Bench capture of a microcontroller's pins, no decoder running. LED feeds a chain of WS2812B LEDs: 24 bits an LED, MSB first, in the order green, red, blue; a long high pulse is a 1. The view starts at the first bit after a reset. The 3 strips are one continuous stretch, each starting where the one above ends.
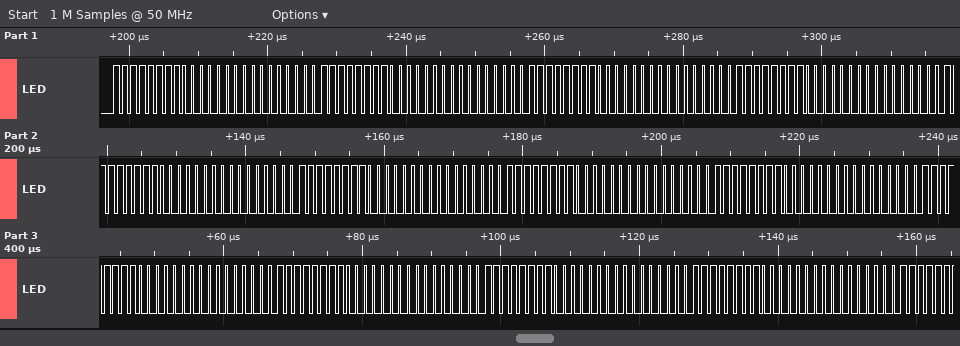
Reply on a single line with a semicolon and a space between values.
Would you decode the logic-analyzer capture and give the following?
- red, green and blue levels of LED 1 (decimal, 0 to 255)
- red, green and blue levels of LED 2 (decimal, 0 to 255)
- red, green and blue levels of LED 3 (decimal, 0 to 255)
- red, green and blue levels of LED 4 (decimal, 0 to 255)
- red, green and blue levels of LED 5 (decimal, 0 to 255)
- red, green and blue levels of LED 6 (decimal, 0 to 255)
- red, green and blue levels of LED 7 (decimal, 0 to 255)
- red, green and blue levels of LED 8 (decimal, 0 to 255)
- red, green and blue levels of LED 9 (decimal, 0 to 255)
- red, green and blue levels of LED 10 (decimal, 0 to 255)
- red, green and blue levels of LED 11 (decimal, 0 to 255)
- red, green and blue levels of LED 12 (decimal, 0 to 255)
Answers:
0, 255, 0; 0, 255, 0; 0, 255, 0; 0, 255, 0; 0, 255, 0; 0, 255, 0; 0, 255, 0; 0, 255, 0; 0, 255, 0; 0, 255, 0; 0, 255, 0; 0, 255, 0
